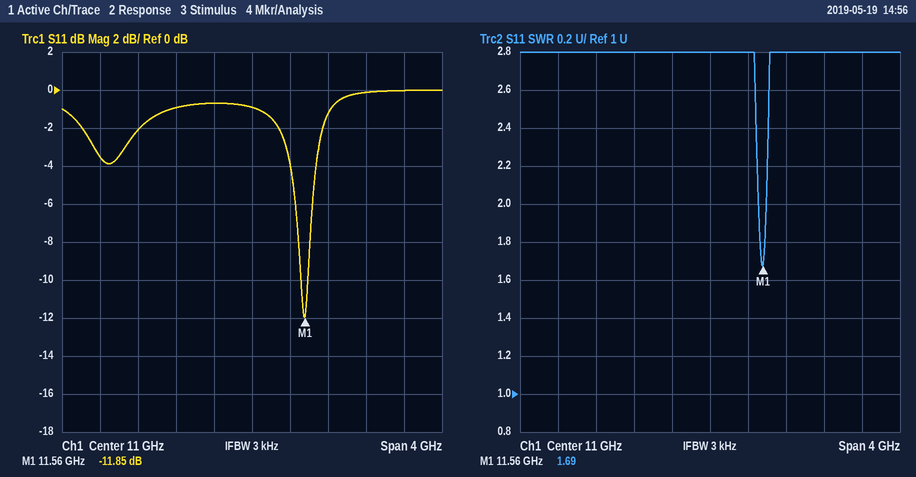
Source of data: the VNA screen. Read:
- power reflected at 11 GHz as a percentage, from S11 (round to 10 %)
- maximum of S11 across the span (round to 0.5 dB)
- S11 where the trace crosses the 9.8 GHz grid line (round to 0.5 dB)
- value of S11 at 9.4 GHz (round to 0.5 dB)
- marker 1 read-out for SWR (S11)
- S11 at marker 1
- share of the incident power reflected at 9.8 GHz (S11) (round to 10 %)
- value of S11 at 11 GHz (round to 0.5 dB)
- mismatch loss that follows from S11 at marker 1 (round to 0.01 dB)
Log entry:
80 %
0.0 dB
-2.0 dB
-3.5 dB
1.69
-11.85 dB
60 %
-1.0 dB
0.29 dB
